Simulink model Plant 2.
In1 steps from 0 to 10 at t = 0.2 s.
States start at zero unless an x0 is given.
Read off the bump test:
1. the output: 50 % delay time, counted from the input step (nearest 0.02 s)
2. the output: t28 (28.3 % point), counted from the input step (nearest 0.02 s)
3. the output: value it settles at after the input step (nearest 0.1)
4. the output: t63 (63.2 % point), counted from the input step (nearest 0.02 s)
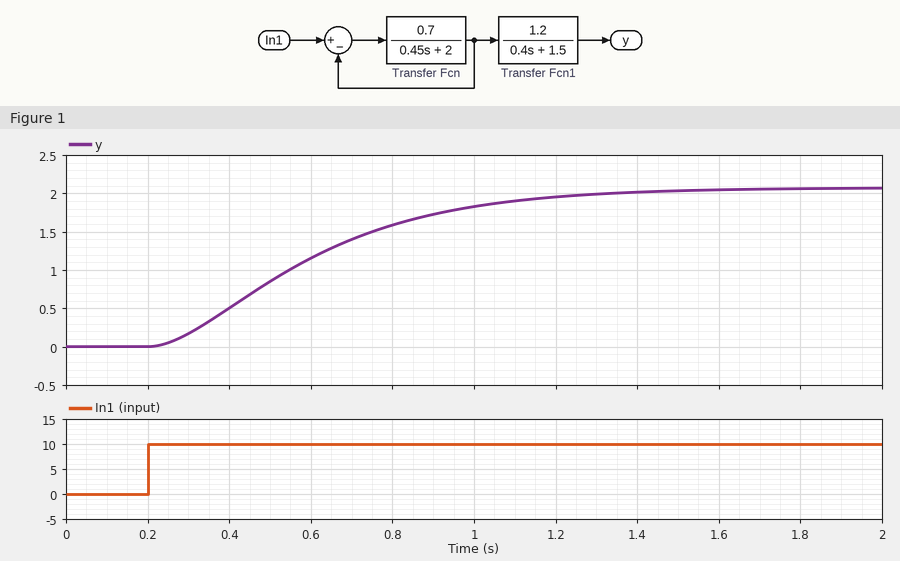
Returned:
0.36 s
0.22 s
2.1
0.46 s
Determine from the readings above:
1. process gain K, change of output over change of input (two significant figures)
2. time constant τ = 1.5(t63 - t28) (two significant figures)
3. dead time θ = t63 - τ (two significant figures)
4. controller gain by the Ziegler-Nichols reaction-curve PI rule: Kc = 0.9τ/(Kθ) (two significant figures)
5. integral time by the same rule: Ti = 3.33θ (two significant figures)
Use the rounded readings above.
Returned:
0.21
0.36 s
0.10 s
15
0.33 s
